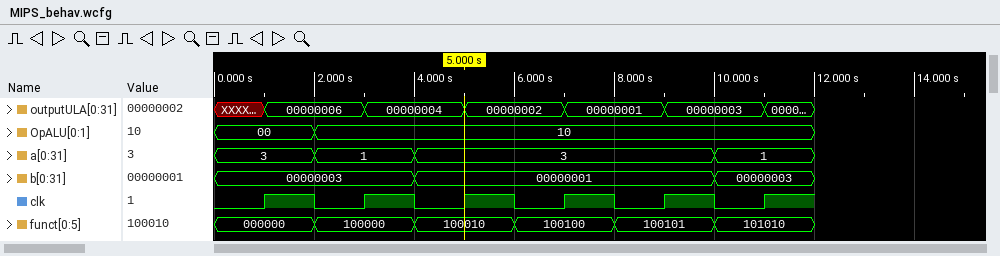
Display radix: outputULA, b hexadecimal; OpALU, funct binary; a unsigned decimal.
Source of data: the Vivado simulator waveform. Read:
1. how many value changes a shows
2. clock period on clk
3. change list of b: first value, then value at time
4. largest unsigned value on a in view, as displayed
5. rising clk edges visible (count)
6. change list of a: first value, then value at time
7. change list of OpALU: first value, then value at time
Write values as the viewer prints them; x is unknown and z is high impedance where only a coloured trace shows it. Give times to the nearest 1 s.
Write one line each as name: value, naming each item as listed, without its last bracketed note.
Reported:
how many value changes a shows: 3
clock period on clk: 2 s
change list of b: first value, then value at time: 00000003, 00000001 at 4 s, 00000003 at 10 s
largest unsigned value on a in view, as displayed: 3
rising clk edges visible: 6
change list of a: first value, then value at time: 3, 1 at 2 s, 3 at 4 s, 1 at 10 s
change list of OpALU: first value, then value at time: 00, 10 at 2 s
